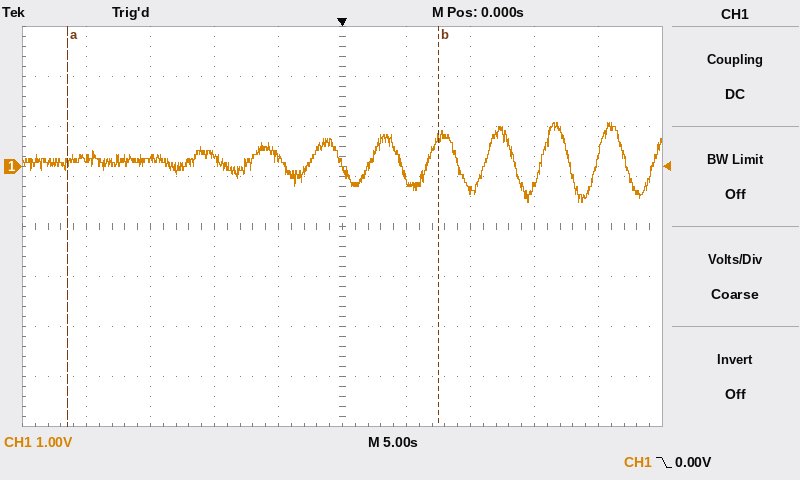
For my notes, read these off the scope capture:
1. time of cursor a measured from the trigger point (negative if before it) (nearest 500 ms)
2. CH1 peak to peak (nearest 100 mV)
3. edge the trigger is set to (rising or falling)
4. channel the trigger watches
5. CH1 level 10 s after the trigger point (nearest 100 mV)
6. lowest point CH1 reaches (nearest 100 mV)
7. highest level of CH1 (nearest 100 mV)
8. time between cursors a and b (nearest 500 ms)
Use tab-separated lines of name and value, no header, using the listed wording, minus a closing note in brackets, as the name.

time of cursor a measured from the trigger point (negative if before it)	-21.5 s
CH1 peak to peak	1.6 V
edge the trigger is set to	falling
channel the trigger watches	CH1
CH1 level 10 s after the trigger point	-500 mV
lowest point CH1 reaches	-700 mV
highest level of CH1	900 mV
time between cursors a and b	29.0 s
